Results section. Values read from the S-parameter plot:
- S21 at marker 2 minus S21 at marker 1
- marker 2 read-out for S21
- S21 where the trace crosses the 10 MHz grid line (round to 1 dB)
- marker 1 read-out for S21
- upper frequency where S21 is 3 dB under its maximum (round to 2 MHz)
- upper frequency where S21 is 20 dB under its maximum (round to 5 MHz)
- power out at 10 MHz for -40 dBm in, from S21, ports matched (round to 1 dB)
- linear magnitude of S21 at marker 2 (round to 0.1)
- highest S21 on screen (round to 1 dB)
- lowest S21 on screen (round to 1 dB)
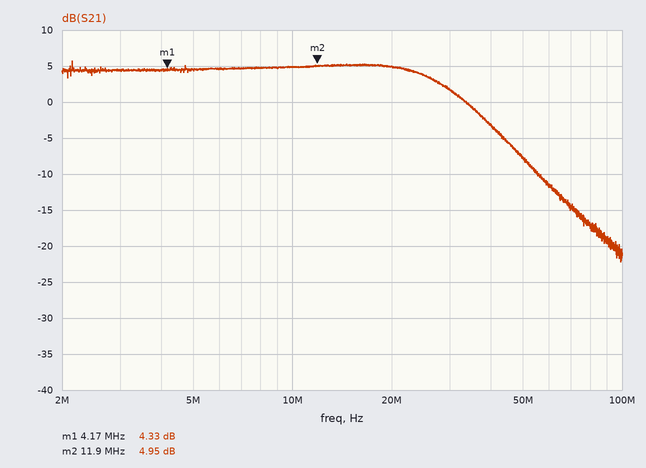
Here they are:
0.62 dB
4.95 dB
5 dB
4.33 dB
28 MHz
70 MHz
-35 dBm
1.8
6 dB
-22 dB
